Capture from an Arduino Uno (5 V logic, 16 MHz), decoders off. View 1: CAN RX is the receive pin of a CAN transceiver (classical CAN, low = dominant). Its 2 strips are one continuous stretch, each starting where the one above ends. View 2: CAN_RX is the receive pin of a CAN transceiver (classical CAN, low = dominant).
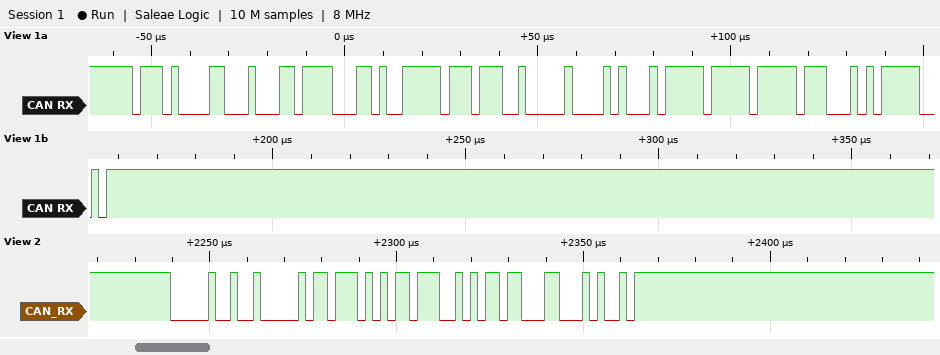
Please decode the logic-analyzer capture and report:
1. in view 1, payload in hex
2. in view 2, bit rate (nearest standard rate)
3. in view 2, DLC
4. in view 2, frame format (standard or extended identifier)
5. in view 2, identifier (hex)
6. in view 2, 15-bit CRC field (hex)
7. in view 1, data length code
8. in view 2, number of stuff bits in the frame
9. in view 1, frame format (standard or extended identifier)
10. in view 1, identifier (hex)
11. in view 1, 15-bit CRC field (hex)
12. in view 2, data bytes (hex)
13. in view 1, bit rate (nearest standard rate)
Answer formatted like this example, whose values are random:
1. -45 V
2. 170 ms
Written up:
1. DE 34 FF 72 00 A2 FF FF
2. 500 kbit/s
3. 3
4. standard
5. 0x012
6. 0x6314
7. 8
8. 2
9. standard
10. 0x743
11. 0x62BE
12. 75 6E 56
13. 500 kbit/s
